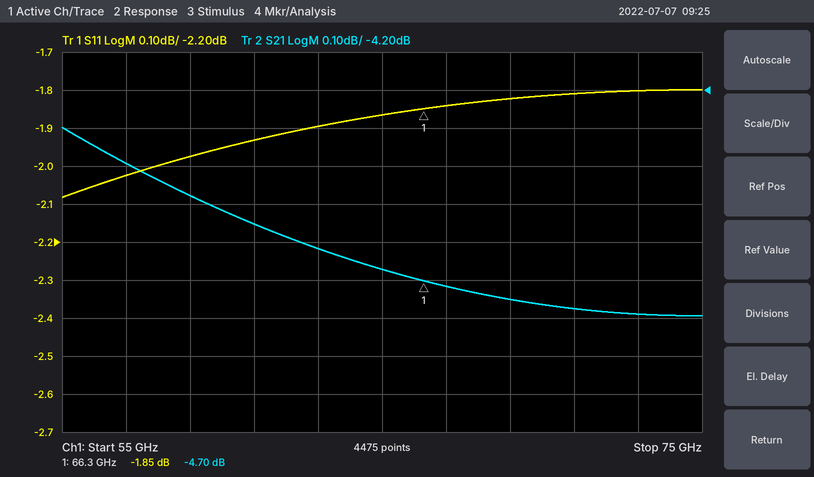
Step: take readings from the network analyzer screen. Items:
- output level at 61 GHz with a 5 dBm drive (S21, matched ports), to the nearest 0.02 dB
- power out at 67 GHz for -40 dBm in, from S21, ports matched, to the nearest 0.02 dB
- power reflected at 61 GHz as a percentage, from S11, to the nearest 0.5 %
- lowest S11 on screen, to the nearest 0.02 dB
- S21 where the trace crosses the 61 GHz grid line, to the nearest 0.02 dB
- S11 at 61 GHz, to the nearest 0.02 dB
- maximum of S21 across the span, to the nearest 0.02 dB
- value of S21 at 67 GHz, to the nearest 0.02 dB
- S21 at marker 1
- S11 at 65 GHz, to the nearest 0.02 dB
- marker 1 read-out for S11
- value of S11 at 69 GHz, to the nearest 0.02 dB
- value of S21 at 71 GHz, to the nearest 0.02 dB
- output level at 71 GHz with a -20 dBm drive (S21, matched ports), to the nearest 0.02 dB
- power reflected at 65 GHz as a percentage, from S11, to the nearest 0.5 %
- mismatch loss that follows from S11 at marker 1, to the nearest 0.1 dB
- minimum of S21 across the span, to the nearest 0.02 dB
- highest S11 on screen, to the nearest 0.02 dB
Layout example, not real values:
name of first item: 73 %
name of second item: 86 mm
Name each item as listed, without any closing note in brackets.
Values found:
output level at 61 GHz with a 5 dBm drive (S21, matched ports), to the nearest 0.02 dB: 0.44 dBm
power out at 67 GHz for -40 dBm in, from S21, ports matched, to the nearest 0.02 dB: -44.72 dBm
power reflected at 61 GHz as a percentage, from S11, to the nearest 0.5 %: 64.0 %
lowest S11 on screen, to the nearest 0.02 dB: -2.08 dB
S21 where the trace crosses the 61 GHz grid line, to the nearest 0.02 dB: -4.56 dB
S11 at 61 GHz, to the nearest 0.02 dB: -1.94 dB
maximum of S21 across the span, to the nearest 0.02 dB: -4.30 dB
value of S21 at 67 GHz, to the nearest 0.02 dB: -4.72 dB
S21 at marker 1: -4.70 dB
S11 at 65 GHz, to the nearest 0.02 dB: -1.86 dB
marker 1 read-out for S11: -1.85 dB
value of S11 at 69 GHz, to the nearest 0.02 dB: -1.82 dB
value of S21 at 71 GHz, to the nearest 0.02 dB: -4.78 dB
output level at 71 GHz with a -20 dBm drive (S21, matched ports), to the nearest 0.02 dB: -24.78 dBm
power reflected at 65 GHz as a percentage, from S11, to the nearest 0.5 %: 65.0 %
mismatch loss that follows from S11 at marker 1, to the nearest 0.1 dB: 4.6 dB
minimum of S21 across the span, to the nearest 0.02 dB: -4.80 dB
highest S11 on screen, to the nearest 0.02 dB: -1.80 dB
